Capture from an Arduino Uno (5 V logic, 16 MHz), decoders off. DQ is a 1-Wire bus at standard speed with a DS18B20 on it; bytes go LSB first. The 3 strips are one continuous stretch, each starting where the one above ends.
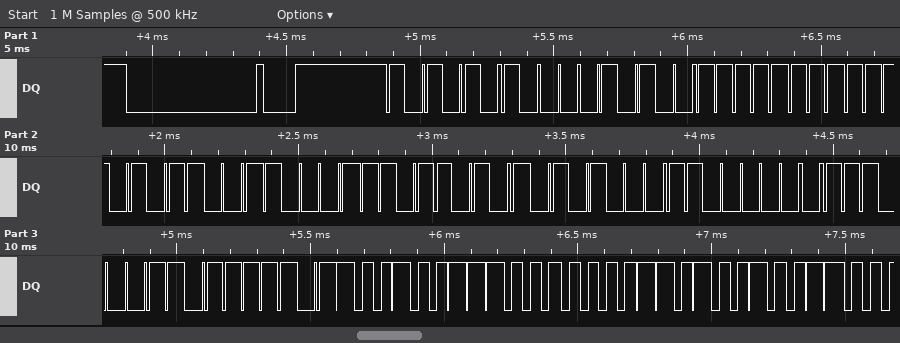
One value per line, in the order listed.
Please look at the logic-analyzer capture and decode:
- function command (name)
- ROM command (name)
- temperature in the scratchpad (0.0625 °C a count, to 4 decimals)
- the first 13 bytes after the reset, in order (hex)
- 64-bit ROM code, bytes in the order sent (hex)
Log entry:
Read Scratchpad
Match ROM
28.5625 °C
55 28 FF D7 8C 5B 15 03 C7 BE C9 01 4B
28 FF D7 8C 5B 15 03 C7
